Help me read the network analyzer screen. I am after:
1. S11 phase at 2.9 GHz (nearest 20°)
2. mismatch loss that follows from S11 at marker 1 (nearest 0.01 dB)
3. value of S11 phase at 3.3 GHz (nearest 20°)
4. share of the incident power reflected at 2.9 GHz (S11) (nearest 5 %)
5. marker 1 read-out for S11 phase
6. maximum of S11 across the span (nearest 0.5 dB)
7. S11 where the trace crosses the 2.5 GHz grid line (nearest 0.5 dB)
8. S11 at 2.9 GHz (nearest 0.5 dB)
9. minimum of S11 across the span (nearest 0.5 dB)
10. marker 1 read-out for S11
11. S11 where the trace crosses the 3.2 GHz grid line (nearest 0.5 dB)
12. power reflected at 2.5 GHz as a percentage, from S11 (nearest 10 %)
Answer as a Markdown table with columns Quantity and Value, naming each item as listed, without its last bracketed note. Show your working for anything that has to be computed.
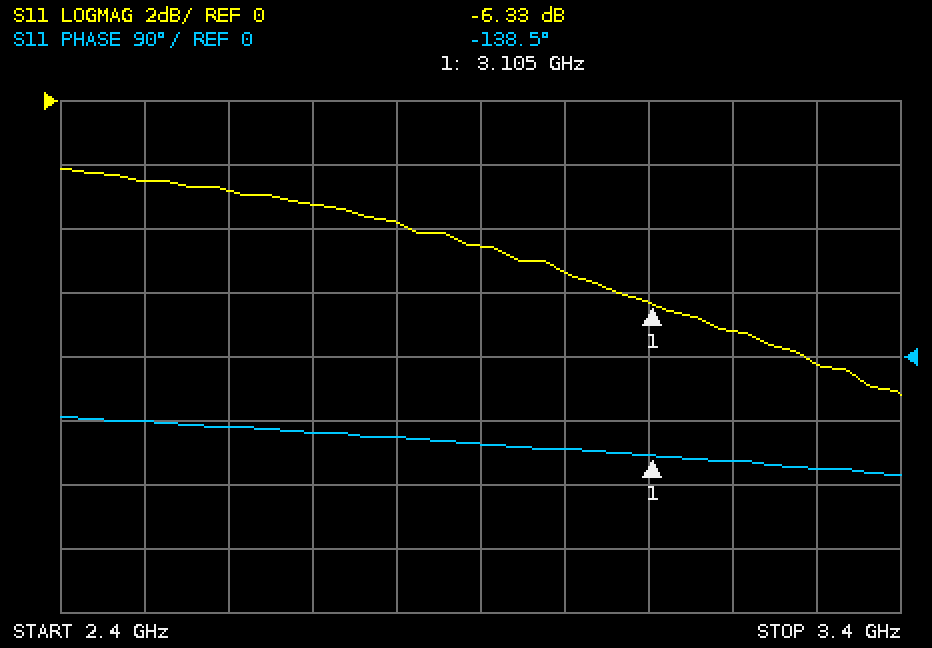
| Quantity | Value |
|---|---|
| S11 phase at 2.9 GHz | -120° |
| mismatch loss that follows from S11 at marker 1 | −10 log10(1 − 10^(-6.33/10)) ≈ 1.15 dB |
| value of S11 phase at 3.3 GHz | -160° |
| share of the incident power reflected at 2.9 GHz (S11) | 10^(-4.5/10) ≈ 35 % |
| marker 1 read-out for S11 phase | -138.5° |
| maximum of S11 across the span | -2.0 dB |
| S11 where the trace crosses the 2.5 GHz grid line | -2.5 dB |
| S11 at 2.9 GHz | -4.5 dB |
| minimum of S11 across the span | -9.0 dB |
| marker 1 read-out for S11 | -6.33 dB |
| S11 where the trace crosses the 3.2 GHz grid line | -7.0 dB |
| power reflected at 2.5 GHz as a percentage, from S11 | 10^(-2.5/10) ≈ 56.2 %, so 60 % to the nearest 10 % |
